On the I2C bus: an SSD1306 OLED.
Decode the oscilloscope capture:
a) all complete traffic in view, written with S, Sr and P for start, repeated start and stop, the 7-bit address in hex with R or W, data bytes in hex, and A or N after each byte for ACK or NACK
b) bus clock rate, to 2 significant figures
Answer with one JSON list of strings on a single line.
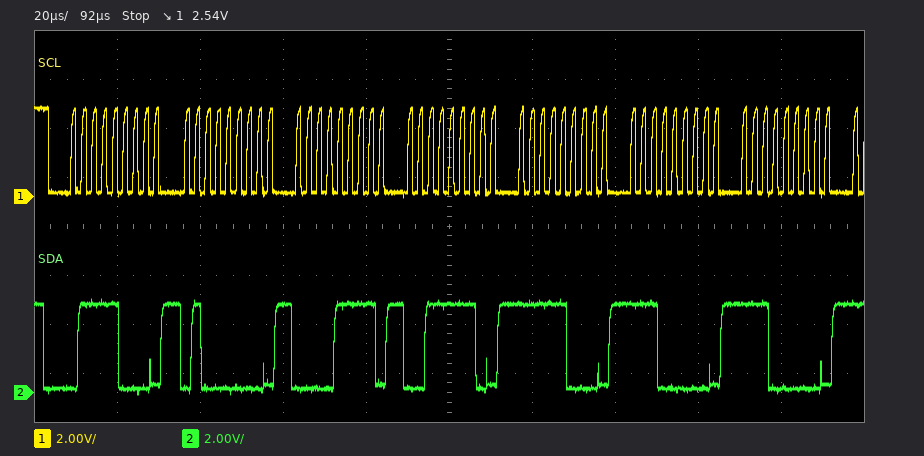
["S 3CW A 40 A 0F A 3E A F8 A E0 A E0 A", "400 kHz"]
